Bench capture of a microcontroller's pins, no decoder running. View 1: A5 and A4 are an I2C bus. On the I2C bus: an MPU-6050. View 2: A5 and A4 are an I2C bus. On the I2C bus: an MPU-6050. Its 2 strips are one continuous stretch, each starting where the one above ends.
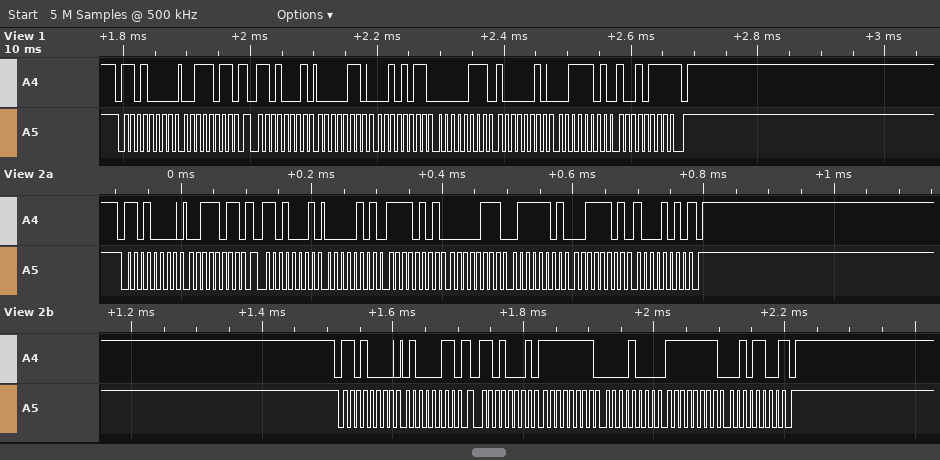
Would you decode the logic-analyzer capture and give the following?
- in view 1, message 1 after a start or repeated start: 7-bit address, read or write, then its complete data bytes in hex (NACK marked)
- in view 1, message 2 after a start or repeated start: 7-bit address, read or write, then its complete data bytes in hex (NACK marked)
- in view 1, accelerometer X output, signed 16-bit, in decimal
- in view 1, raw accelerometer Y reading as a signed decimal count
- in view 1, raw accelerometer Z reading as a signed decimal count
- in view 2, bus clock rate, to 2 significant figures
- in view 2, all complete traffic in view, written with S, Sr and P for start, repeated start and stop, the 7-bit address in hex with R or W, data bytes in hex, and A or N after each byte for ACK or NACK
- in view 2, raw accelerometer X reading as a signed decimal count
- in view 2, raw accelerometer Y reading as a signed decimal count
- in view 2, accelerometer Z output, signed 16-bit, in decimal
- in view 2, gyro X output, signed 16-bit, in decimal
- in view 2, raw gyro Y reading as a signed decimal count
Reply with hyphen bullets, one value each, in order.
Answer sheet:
- 0x68 write: 3B
- 0x68 read: 06 2B 07 82 3D 97 NACK
- 1579
- 1922
- 15767
- 100 kHz
- S 68W A 3B A Sr 68R A 05 A F5 A 07 A 7D A 3D A 8A N P S 68W A 43 A Sr 68R A FF A 08 A FF A 2C N P
- 1525
- 1917
- 15754
- -248
- -212
